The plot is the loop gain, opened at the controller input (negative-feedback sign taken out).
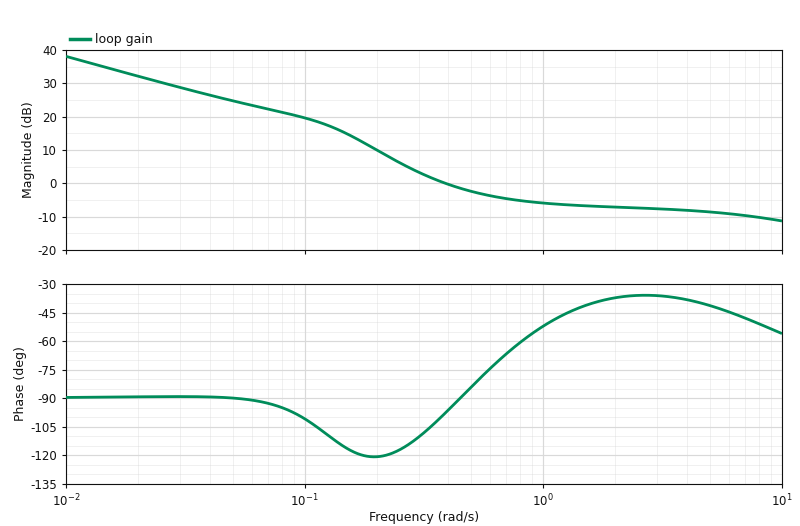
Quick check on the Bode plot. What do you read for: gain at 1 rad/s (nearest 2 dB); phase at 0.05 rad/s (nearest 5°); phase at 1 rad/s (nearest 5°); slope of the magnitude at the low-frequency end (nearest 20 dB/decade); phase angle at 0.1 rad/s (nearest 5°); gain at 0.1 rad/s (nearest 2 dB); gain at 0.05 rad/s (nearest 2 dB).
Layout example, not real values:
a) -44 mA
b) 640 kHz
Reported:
a) -6 dB
b) -90°
c) -50°
d) -20 dB/decade
e) -100°
f) 20 dB
g) 24 dB
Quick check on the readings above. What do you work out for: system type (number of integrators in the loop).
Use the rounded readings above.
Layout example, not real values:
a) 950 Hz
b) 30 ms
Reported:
a) 1
